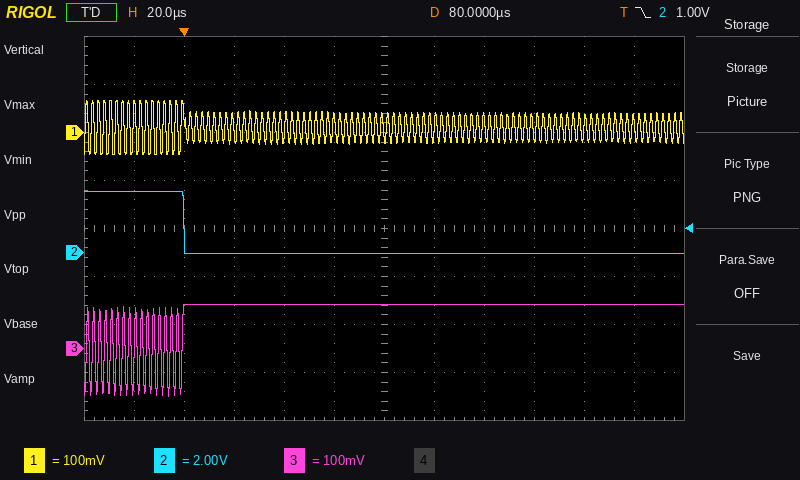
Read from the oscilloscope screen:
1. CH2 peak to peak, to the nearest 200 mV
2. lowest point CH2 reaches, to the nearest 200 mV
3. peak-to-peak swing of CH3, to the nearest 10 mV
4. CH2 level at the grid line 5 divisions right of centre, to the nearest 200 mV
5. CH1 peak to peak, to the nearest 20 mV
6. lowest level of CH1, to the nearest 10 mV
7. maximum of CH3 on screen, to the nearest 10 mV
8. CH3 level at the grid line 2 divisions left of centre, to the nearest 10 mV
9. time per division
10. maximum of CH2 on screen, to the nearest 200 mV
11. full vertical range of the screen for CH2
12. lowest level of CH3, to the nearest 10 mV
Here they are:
2.6 V
0.0 V
190 mV
0.0 V
120 mV
-50 mV
90 mV
90 mV
20 µs
2.6 V
16 V
-100 mV
